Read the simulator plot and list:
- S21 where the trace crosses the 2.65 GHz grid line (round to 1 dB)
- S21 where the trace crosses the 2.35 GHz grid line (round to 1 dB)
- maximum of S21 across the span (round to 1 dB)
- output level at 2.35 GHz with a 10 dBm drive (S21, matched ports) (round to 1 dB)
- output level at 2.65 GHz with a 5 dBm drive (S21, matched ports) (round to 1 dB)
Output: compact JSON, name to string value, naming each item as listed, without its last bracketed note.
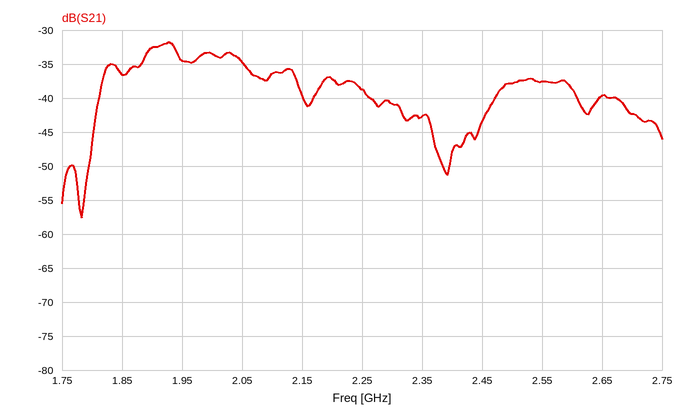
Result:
{"S21 where the trace crosses the 2.65 GHz grid line": "-40 dB", "S21 where the trace crosses the 2.35 GHz grid line": "-43 dB", "maximum of S21 across the span": "-32 dB", "output level at 2.35 GHz with a 10 dBm drive (S21, matched ports)": "-33 dBm", "output level at 2.65 GHz with a 5 dBm drive (S21, matched ports)": "-35 dBm"}
